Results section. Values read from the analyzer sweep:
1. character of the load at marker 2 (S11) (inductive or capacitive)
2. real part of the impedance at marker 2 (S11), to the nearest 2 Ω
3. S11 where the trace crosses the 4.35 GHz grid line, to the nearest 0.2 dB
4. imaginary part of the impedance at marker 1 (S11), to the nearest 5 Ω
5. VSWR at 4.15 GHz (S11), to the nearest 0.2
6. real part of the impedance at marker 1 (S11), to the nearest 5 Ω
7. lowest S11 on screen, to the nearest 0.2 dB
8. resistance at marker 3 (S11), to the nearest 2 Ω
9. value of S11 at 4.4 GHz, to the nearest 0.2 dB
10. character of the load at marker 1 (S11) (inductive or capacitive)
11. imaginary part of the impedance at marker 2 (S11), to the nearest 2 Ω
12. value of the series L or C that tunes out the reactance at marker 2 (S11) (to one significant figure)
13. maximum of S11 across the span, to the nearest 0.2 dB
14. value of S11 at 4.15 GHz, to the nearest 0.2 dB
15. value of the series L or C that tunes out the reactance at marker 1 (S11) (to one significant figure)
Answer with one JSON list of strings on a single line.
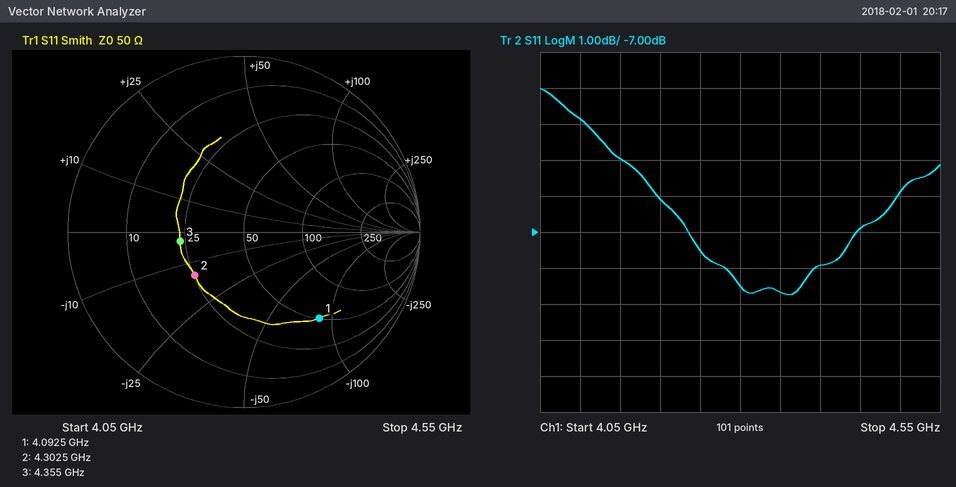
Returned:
["capacitive", "26 Ω", "-8.6 dB", "-85 Ω", "3.6", "50 Ω", "-8.8 dB", "24 Ω", "-8.0 dB", "capacitive", "-14 Ω", "500 pH", "-3.0 dB", "-5.0 dB", "3 nH"]
